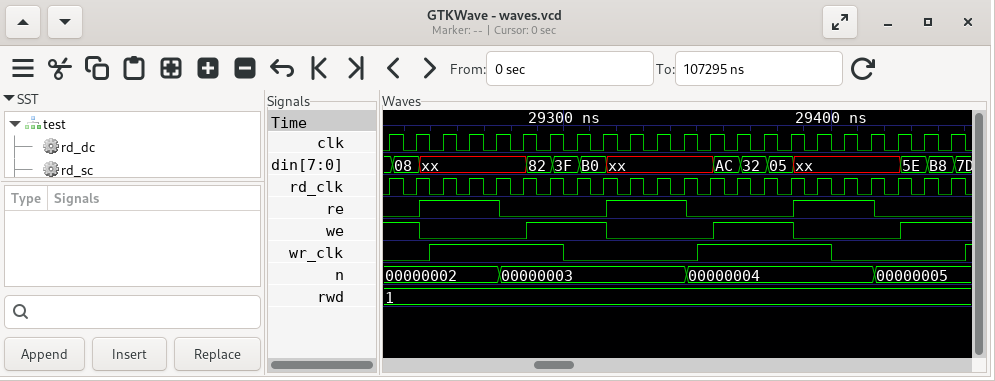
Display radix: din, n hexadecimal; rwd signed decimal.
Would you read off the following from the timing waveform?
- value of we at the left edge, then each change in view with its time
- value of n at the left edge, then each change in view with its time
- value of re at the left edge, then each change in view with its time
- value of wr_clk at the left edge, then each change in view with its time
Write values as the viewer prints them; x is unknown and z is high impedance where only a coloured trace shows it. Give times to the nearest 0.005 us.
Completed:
1, 0 at 29.245 us, 1 at 29.285 us, 0 at 29.315 us, 1 at 29.355 us, 0 at 29.385 us, 1 at 29.425 us
00000002, 00000003 at 29.275 us, 00000004 at 29.345 us, 00000005 at 29.415 us
0, 1 at 29.245 us, 0 at 29.275 us, 1 at 29.315 us, 0 at 29.345 us, 1 at 29.385 us, 0 at 29.415 us
0, 1 at 29.25 us, 0 at 29.3 us, 1 at 29.35 us, 0 at 29.4 us, 1 at 29.45 us
